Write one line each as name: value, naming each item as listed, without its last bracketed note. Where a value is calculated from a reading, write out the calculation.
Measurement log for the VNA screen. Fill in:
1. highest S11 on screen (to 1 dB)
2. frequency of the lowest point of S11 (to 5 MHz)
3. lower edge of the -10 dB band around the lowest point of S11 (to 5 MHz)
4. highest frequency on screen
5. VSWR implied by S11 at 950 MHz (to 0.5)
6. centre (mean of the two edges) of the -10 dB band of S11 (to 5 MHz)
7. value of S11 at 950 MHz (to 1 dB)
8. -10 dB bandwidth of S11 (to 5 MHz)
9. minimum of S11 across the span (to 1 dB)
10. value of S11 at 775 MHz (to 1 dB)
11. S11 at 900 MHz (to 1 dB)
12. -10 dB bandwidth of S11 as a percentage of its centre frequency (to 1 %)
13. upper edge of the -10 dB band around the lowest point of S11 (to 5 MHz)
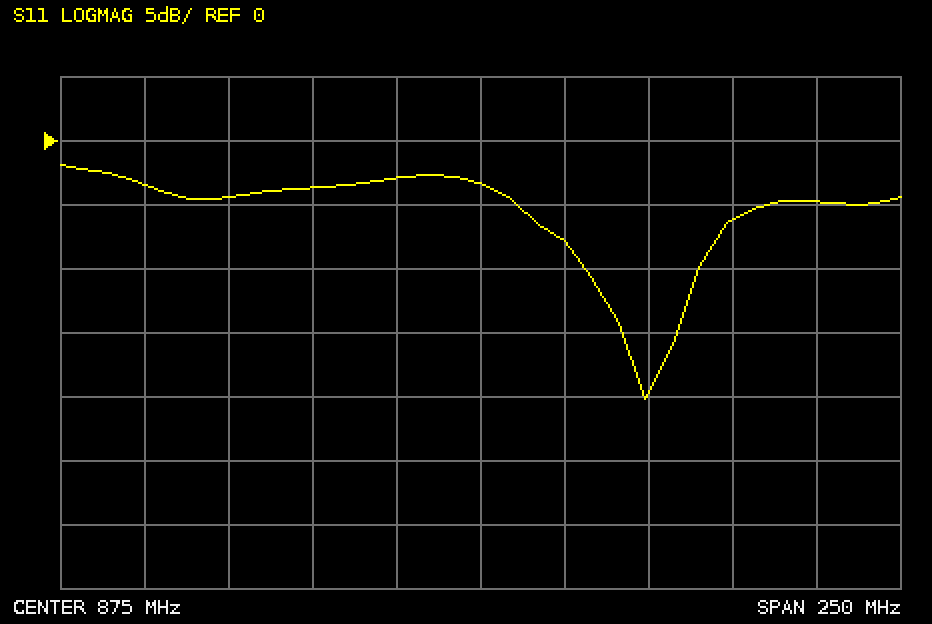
highest S11 on screen: -2 dB
frequency of the lowest point of S11: 925 MHz
lower edge of the -10 dB band around the lowest point of S11: 905 MHz
highest frequency on screen: 1 GHz
VSWR implied by S11 at 950 MHz: |Γ| = 10^(-6/20) = 0.5012; VSWR = (1 + 0.5012)/(1 − 0.5012) ≈ 3.0
centre (mean of the two edges) of the -10 dB band of S11: 925 MHz
value of S11 at 950 MHz: -6 dB
-10 dB bandwidth of S11: 940 MHz − 905 MHz = 35 MHz
minimum of S11 across the span: -20 dB
value of S11 at 775 MHz: -3 dB
S11 at 900 MHz: -8 dB
-10 dB bandwidth of S11 as a percentage of its centre frequency: 35 MHz / 922.5 MHz ≈ 4 %
upper edge of the -10 dB band around the lowest point of S11: 940 MHz
